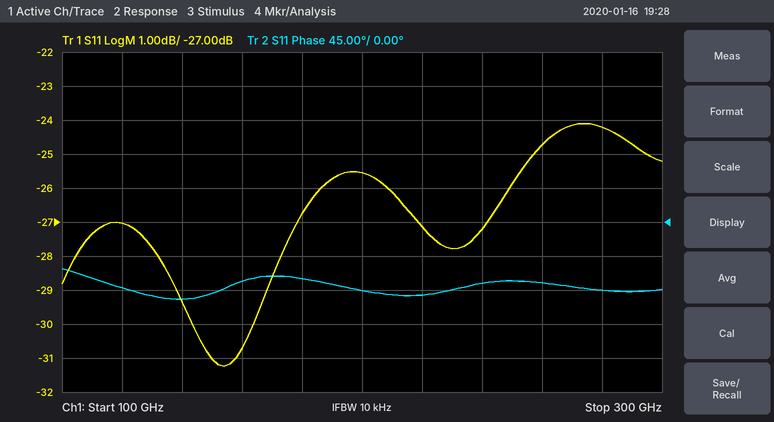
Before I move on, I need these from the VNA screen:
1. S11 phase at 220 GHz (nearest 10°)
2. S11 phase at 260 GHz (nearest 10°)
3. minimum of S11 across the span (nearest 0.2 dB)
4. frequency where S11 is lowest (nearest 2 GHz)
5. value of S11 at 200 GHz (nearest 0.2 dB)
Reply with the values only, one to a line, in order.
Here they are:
-100°
-80°
-31.2 dB
154 GHz
-25.6 dB
